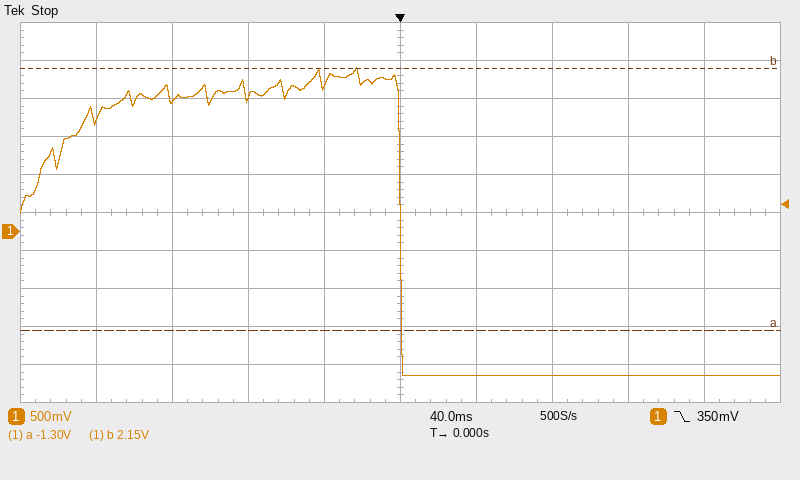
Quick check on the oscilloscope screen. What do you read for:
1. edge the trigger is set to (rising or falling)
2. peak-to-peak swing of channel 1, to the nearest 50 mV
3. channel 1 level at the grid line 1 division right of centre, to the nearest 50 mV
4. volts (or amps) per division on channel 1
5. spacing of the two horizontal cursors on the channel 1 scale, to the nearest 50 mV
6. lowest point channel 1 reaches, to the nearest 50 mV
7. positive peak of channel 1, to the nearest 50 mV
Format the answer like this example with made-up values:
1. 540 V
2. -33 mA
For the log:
1. falling
2. 4.05 V
3. -1.90 V
4. 500 mV
5. 3.45 V
6. -1.90 V
7. 2.15 V
